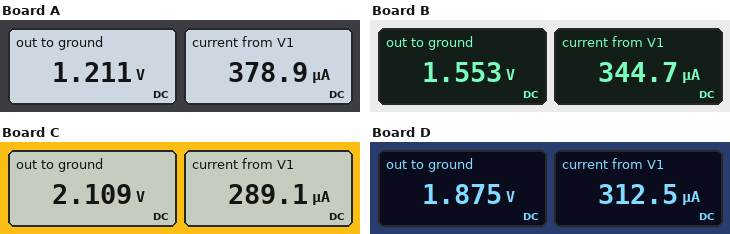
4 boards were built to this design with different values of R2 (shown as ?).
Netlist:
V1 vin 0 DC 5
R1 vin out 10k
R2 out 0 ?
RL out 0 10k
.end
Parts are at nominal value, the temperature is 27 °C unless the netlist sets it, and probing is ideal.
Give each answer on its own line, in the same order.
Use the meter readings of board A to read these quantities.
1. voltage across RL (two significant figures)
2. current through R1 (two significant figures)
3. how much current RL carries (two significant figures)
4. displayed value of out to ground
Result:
1.2 V
380 µA
120 µA
1.211 V
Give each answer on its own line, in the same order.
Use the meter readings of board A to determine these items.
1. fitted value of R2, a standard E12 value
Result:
4.7 kΩ
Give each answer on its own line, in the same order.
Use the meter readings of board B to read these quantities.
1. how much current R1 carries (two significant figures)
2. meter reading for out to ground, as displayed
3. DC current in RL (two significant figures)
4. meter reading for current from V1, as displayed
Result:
340 µA
1.553 V
160 µA
344.7 µA
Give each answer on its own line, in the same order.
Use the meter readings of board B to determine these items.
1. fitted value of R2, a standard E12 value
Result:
8.2 kΩ
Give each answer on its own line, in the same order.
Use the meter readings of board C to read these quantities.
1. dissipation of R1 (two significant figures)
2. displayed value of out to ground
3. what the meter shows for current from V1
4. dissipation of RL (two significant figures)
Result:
840 µW
2.109 V
289.1 µA
440 µW
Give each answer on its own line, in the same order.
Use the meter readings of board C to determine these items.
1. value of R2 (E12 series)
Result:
27 kΩ
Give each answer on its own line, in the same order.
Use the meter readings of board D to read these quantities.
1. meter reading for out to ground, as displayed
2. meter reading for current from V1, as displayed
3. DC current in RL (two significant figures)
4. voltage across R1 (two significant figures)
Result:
1.875 V
312.5 µA
190 µA
3.1 V
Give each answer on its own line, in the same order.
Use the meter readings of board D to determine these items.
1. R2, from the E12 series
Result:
15 kΩ
